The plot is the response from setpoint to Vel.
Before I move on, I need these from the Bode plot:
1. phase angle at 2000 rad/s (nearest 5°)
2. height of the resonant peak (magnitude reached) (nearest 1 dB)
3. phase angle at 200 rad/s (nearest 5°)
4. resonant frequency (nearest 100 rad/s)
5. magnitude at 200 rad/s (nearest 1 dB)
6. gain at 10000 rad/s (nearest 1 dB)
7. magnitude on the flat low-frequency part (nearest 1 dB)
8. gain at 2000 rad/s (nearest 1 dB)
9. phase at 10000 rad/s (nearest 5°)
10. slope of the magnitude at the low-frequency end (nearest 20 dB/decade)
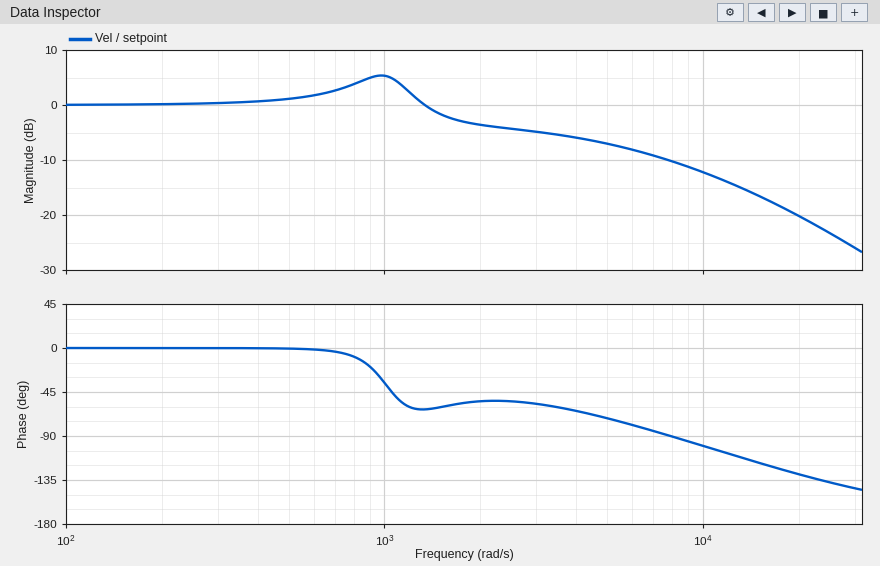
-55°
5 dB
0°
1000 rad/s
0 dB
-12 dB
0 dB
-4 dB
-100°
0 dB/decade
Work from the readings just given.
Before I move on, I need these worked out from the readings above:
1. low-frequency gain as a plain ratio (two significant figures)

1.0
